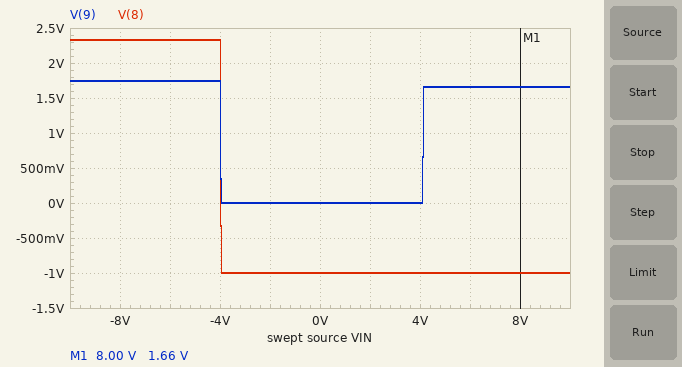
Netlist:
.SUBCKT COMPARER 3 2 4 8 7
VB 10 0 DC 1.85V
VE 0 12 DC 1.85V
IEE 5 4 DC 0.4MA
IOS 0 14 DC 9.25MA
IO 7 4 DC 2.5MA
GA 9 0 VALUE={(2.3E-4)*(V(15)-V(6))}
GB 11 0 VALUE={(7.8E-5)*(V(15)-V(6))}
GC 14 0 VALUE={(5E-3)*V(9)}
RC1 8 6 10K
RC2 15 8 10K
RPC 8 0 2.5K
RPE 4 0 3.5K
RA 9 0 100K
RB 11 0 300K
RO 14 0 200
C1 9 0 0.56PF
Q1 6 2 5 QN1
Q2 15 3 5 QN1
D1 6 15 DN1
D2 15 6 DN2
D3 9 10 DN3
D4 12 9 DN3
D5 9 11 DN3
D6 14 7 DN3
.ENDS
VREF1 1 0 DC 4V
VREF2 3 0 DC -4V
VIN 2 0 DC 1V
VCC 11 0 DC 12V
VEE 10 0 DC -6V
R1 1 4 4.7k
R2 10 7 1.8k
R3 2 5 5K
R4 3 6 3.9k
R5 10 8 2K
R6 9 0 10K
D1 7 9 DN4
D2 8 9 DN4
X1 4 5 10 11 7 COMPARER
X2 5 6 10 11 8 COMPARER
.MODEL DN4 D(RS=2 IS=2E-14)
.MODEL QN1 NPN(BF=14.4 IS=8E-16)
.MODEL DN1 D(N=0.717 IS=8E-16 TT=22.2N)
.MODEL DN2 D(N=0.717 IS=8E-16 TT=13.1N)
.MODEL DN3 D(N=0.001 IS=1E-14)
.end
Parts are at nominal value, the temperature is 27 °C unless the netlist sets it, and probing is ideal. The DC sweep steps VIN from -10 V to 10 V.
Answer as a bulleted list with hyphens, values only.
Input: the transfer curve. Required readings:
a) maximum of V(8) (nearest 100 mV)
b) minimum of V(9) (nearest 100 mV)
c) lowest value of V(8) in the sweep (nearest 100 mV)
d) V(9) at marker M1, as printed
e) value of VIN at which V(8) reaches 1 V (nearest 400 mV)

- 2.3 V
- 0 V
- -1.0 V
- 1.66 V
- -4.0 V
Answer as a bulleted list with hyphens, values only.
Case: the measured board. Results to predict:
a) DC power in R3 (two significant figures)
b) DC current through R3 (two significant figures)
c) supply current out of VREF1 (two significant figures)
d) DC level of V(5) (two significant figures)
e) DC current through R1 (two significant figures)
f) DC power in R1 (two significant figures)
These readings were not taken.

- 3.4 µW
- 26 µA
- 26 µA
- 870 mV
- 26 µA
- 3.2 µW
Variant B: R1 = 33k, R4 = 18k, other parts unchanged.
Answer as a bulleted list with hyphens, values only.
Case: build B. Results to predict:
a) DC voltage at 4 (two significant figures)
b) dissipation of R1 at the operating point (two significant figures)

- 3.1 V
- 22 µW
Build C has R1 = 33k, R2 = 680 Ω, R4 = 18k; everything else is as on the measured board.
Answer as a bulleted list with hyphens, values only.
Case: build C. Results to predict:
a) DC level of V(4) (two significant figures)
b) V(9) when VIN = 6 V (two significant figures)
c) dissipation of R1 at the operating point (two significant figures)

- 3.1 V
- 540 mV
- 22 µW
